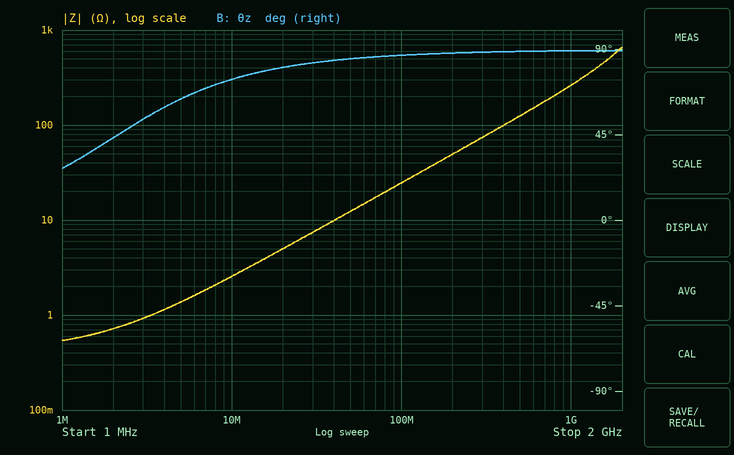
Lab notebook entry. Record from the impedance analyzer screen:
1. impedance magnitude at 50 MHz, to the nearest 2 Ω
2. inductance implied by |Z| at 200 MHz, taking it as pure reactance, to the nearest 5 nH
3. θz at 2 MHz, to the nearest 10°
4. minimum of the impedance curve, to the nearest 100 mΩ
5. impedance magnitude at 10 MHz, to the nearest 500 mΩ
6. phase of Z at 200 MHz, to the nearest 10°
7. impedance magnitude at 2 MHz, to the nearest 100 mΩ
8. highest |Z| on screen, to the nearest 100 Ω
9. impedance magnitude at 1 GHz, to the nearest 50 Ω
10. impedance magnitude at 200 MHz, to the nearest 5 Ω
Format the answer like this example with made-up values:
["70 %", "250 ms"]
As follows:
["12 Ω", "40 nH", "40°", "500 mΩ", "2.5 Ω", "90°", "700 mΩ", "700 Ω", "250 Ω", "50 Ω"]
